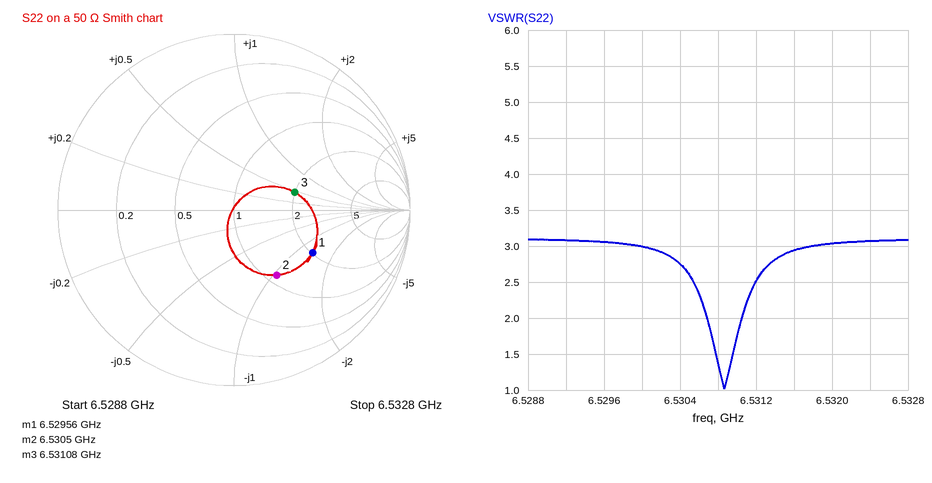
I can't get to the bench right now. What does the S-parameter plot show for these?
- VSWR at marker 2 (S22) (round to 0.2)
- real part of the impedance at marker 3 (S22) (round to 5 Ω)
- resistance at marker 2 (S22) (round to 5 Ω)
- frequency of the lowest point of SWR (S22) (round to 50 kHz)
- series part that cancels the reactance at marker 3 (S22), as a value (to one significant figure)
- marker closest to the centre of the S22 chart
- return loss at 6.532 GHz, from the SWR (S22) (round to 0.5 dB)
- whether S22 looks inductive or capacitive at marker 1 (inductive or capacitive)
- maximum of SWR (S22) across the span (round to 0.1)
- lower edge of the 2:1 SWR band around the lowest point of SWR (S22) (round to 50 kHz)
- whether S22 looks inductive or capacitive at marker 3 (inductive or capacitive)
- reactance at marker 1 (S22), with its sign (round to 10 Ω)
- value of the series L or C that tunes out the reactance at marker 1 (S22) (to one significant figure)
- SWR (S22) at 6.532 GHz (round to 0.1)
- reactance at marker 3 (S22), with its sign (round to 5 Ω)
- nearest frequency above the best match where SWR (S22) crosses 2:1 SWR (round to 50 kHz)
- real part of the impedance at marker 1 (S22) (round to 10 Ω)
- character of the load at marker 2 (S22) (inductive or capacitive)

2.6
100 Ω
55 Ω
6.53085 GHz
1 pF
marker 3
6.0 dB
capacitive
3.1
6.53070 GHz
inductive
-70 Ω
2 nH
3.0
+25 Ω
6.53105 GHz
100 Ω
capacitive
